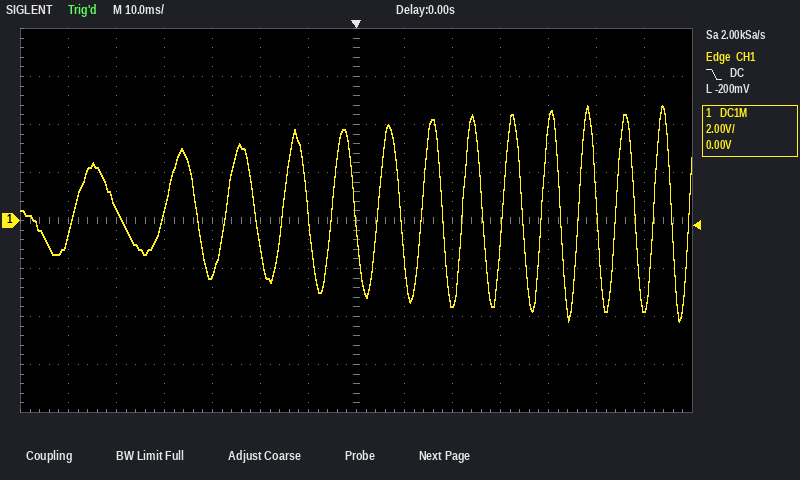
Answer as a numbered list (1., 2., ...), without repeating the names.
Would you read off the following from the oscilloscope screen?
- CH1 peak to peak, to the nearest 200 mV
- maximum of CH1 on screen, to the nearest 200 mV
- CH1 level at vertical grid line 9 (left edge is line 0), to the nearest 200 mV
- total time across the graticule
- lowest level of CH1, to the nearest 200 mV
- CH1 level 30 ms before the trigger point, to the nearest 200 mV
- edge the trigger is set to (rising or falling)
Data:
1. 9.0 V
2. 4.8 V
3. -3.4 V
4. 140 ms
5. -4.2 V
6. -2.2 V
7. falling
